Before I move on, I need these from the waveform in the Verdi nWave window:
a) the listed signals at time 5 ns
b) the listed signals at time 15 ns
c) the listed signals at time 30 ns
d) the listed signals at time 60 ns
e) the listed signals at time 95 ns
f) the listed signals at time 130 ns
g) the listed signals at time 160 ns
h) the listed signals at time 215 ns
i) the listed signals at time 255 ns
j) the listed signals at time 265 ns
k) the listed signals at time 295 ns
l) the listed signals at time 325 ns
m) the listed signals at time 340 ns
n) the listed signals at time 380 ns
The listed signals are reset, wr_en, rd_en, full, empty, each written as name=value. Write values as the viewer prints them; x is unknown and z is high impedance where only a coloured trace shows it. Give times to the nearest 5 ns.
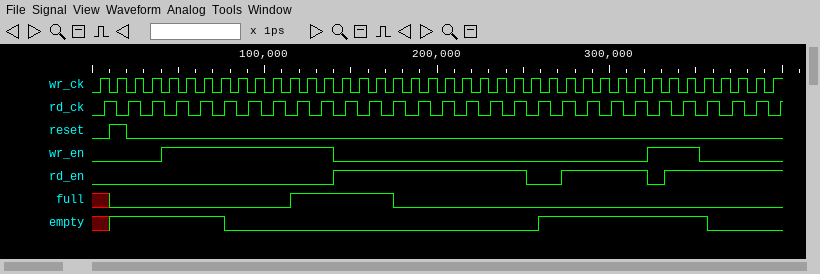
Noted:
reset=0, wr_en=0, rd_en=0, full=x, empty=x
reset=1, wr_en=0, rd_en=0, full=0, empty=1
reset=0, wr_en=0, rd_en=0, full=0, empty=1
reset=0, wr_en=1, rd_en=0, full=0, empty=1
reset=0, wr_en=1, rd_en=0, full=0, empty=0
reset=0, wr_en=1, rd_en=0, full=1, empty=0
reset=0, wr_en=0, rd_en=1, full=1, empty=0
reset=0, wr_en=0, rd_en=1, full=0, empty=0
reset=0, wr_en=0, rd_en=0, full=0, empty=0
reset=0, wr_en=0, rd_en=0, full=0, empty=1
reset=0, wr_en=0, rd_en=1, full=0, empty=1
reset=0, wr_en=1, rd_en=0, full=0, empty=1
reset=0, wr_en=1, rd_en=1, full=0, empty=1
reset=0, wr_en=0, rd_en=1, full=0, empty=0
